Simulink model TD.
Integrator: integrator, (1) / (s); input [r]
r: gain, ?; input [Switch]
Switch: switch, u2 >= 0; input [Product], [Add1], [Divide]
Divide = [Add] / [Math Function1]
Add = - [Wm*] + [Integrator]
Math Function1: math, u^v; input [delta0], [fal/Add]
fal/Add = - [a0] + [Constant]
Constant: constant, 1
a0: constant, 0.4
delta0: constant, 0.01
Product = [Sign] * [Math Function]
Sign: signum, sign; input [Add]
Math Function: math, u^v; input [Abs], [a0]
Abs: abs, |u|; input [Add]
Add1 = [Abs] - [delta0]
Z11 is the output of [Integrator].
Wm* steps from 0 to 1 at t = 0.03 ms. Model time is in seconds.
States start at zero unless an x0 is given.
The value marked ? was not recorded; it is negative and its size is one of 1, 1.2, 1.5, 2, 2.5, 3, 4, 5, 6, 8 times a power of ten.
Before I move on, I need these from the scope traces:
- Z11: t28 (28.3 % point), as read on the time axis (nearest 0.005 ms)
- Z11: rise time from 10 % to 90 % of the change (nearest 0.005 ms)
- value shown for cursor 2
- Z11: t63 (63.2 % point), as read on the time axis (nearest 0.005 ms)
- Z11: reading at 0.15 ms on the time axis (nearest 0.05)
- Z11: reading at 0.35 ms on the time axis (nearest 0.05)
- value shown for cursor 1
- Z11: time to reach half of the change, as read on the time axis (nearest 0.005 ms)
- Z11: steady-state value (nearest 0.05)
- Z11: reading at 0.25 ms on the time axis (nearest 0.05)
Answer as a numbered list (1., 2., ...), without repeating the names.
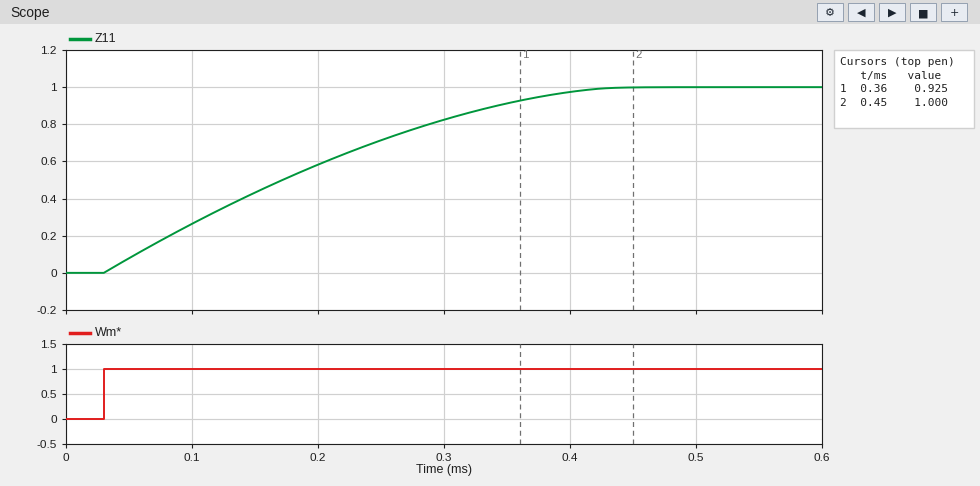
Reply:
1. 0.105 ms
2. 0.285 ms
3. 1.000
4. 0.220 ms
5. 0.45
6. 0.90
7. 0.925
8. 0.170 ms
9. 1.00
10. 0.70
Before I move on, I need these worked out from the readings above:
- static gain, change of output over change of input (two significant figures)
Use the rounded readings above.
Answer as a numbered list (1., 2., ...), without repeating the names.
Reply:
1. 1.0
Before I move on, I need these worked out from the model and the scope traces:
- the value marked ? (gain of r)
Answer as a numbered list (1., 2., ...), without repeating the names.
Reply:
1. -4000
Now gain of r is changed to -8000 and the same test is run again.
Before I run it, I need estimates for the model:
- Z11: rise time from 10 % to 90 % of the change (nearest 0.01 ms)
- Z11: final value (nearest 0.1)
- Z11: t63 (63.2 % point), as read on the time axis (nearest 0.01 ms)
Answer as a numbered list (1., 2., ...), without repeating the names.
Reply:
1. 0.14 ms
2. 1.0
3. 0.12 ms
